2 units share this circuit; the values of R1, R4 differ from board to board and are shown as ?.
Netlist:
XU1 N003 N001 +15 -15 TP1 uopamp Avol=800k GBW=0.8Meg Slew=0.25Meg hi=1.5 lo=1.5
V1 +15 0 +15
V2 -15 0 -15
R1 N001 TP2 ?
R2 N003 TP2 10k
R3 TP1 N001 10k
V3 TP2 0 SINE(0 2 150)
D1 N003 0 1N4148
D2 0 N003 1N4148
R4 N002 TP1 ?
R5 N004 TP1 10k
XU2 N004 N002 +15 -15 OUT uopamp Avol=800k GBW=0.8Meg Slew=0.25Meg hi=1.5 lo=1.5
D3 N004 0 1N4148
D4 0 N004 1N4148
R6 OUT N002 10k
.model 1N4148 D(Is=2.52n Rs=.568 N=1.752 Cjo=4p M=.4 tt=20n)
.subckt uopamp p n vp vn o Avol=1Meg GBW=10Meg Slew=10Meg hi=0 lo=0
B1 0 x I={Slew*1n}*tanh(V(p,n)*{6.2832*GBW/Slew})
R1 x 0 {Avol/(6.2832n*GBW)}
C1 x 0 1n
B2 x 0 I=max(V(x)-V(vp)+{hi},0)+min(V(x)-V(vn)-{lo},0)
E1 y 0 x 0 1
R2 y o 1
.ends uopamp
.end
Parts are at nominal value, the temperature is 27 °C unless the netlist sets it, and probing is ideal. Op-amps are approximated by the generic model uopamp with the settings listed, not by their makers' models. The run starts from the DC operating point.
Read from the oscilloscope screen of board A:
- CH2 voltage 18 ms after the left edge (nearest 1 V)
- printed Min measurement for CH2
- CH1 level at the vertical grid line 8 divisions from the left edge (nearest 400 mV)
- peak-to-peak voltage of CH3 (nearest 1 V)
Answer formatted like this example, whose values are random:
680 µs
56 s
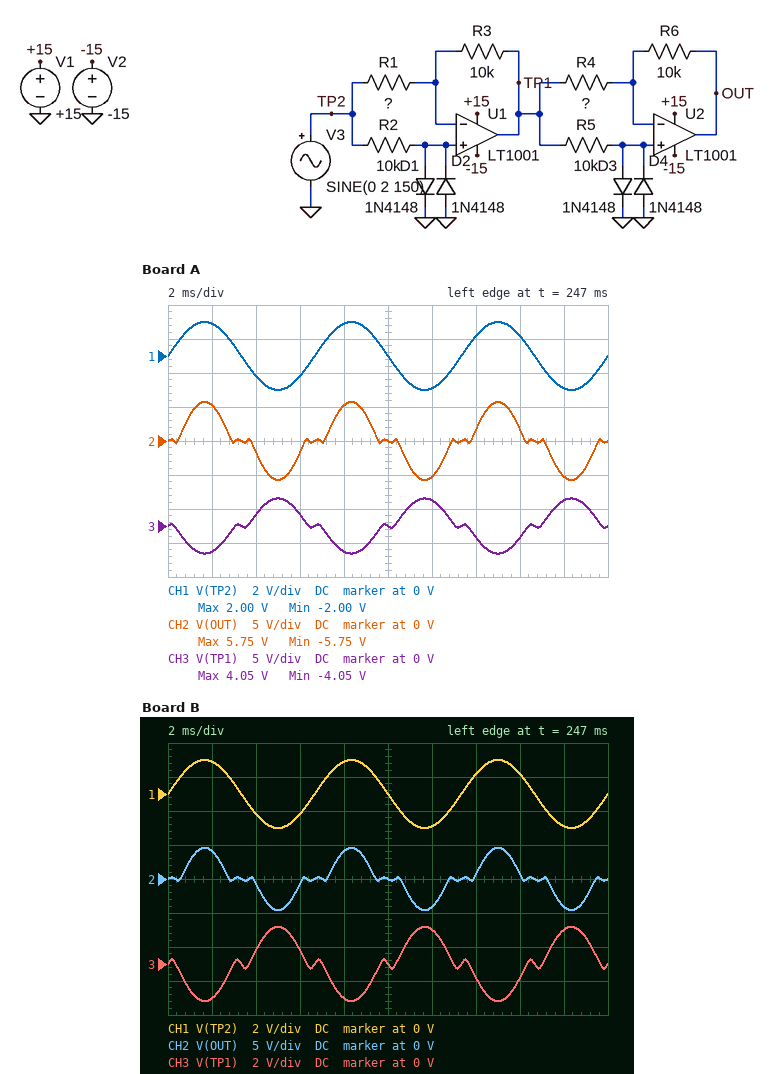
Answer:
-5 V
-5.75 V
1.2 V
8 V
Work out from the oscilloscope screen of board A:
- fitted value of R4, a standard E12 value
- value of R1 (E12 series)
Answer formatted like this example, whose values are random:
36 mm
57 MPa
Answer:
5.6 kΩ
3.3 kΩ
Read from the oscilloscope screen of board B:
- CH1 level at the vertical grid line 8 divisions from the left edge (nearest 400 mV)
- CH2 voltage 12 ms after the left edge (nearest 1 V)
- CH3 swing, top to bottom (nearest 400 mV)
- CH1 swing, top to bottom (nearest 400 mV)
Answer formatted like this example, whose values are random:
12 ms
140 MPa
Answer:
1.2 V
-4 V
4.4 V
4.0 V
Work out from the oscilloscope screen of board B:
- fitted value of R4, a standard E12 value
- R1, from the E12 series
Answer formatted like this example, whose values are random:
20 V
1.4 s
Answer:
3.3 kΩ
5.6 kΩ
